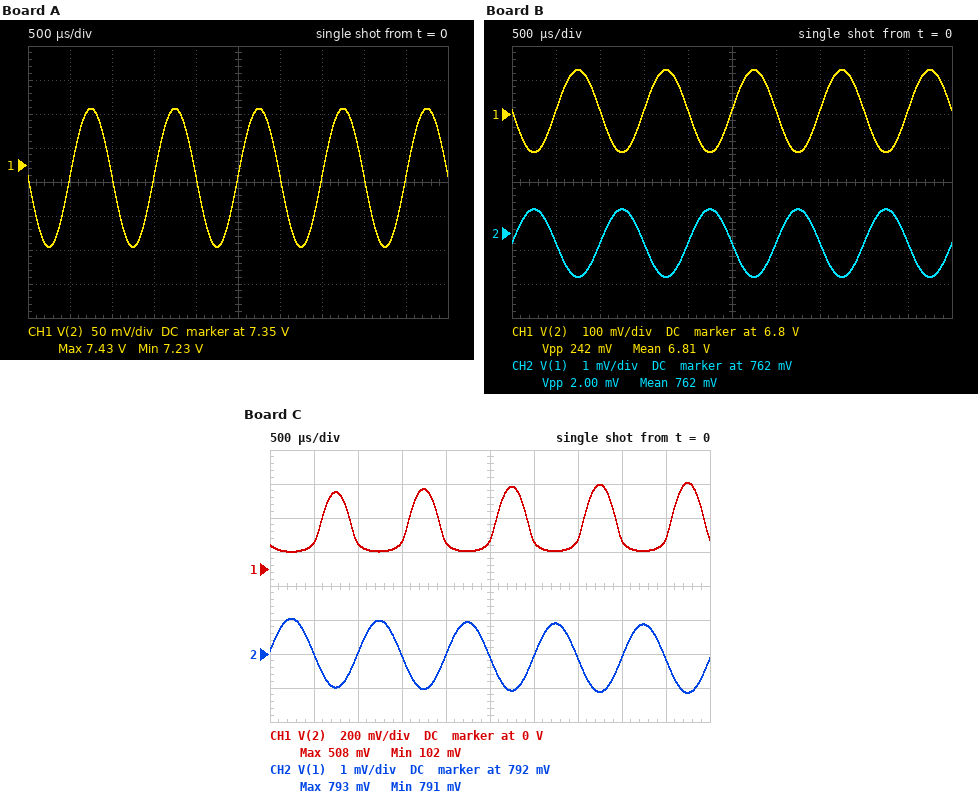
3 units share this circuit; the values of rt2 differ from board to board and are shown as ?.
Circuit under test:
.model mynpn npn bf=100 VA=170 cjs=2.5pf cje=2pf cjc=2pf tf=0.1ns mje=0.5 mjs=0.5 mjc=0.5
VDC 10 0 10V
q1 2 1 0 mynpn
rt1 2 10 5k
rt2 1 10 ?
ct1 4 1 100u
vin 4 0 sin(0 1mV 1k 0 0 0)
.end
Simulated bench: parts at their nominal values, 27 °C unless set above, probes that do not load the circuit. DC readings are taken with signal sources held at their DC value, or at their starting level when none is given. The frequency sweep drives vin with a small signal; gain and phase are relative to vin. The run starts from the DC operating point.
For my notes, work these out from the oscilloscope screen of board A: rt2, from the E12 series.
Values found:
1.8 MΩ
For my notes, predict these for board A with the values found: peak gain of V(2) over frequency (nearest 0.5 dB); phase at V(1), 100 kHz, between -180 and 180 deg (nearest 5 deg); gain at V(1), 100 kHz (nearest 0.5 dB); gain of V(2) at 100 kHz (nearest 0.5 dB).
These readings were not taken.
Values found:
40.0 dB
0 deg
0 dB
40.0 dB
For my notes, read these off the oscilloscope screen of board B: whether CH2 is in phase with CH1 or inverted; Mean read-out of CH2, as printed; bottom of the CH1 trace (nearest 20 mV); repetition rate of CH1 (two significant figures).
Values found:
inverted
762 mV
6.68 V
1.0 kHz
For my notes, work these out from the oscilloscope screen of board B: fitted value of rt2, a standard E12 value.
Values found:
1.5 MΩ
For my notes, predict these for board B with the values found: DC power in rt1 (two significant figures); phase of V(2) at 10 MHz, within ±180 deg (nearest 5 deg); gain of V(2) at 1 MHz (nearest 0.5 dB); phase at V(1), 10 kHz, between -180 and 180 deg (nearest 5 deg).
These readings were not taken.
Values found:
2.0 mW
155 deg
41.5 dB
0 deg
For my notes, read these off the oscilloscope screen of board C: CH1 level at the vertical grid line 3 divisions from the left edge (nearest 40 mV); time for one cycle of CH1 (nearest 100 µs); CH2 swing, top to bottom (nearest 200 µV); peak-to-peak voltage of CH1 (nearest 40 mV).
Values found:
160 mV
1.0 ms
2.2 mV
400 mV
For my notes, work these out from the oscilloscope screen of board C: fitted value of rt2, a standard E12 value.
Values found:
330 kΩ
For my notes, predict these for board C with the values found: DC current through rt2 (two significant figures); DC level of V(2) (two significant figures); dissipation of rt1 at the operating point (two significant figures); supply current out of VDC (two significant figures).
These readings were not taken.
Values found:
28 µA
140 mV
19 mW
2.0 mA
